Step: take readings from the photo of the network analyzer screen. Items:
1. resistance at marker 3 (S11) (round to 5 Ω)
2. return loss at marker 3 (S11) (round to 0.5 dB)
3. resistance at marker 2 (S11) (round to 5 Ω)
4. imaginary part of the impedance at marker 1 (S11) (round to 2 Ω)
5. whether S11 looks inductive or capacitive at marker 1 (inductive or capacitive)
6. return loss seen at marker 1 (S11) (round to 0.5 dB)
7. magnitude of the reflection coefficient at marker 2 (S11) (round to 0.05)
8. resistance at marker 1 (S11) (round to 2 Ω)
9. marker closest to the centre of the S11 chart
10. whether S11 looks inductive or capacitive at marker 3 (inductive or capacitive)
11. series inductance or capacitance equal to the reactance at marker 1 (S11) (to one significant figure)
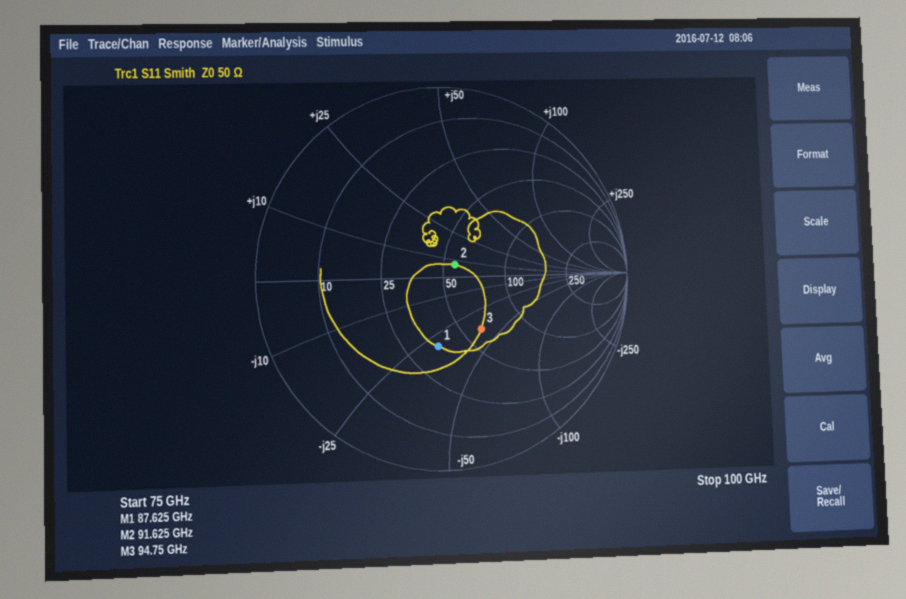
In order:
60 Ω
9.5 dB
55 Ω
-30 Ω
capacitive
9.0 dB
0.10
36 Ω
marker 2
capacitive
60 fF
